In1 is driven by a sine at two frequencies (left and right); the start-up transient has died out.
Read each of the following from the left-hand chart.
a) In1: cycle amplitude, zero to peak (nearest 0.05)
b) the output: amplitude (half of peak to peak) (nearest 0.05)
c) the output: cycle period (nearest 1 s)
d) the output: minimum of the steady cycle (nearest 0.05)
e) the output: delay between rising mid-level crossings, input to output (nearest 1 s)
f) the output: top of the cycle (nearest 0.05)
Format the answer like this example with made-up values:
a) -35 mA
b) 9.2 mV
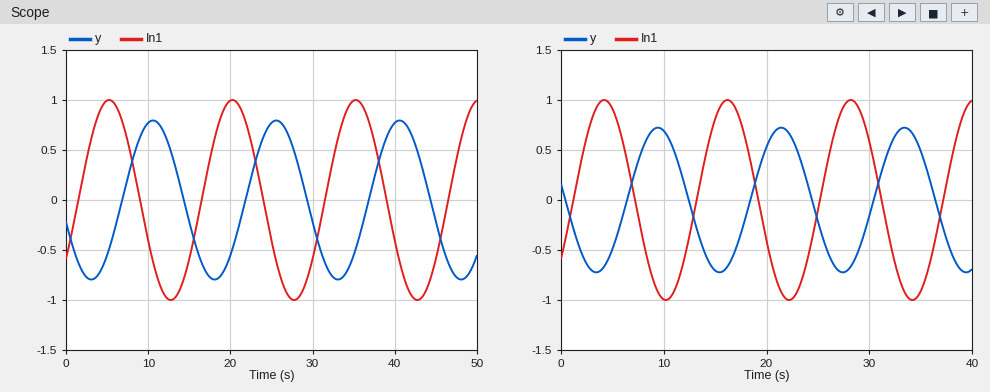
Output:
a) 1.00
b) 0.80
c) 15 s
d) -0.80
e) 5 s
f) 0.80
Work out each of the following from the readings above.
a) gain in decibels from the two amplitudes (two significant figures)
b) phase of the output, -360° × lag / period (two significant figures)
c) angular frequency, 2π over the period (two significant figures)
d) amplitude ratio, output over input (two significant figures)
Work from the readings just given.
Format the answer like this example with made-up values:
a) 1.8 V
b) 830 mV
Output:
a) -1.9 dB
b) -120°
c) 0.42 rad/s
d) 0.80
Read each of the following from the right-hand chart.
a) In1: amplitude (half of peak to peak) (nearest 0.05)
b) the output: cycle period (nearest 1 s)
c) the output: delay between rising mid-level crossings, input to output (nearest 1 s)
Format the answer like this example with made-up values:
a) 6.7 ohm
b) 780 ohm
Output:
a) 1.00
b) 12 s
c) 5 s
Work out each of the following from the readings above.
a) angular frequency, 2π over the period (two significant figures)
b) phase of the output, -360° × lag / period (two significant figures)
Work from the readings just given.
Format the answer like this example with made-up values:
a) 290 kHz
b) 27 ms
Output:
a) 0.52 rad/s
b) -150°
